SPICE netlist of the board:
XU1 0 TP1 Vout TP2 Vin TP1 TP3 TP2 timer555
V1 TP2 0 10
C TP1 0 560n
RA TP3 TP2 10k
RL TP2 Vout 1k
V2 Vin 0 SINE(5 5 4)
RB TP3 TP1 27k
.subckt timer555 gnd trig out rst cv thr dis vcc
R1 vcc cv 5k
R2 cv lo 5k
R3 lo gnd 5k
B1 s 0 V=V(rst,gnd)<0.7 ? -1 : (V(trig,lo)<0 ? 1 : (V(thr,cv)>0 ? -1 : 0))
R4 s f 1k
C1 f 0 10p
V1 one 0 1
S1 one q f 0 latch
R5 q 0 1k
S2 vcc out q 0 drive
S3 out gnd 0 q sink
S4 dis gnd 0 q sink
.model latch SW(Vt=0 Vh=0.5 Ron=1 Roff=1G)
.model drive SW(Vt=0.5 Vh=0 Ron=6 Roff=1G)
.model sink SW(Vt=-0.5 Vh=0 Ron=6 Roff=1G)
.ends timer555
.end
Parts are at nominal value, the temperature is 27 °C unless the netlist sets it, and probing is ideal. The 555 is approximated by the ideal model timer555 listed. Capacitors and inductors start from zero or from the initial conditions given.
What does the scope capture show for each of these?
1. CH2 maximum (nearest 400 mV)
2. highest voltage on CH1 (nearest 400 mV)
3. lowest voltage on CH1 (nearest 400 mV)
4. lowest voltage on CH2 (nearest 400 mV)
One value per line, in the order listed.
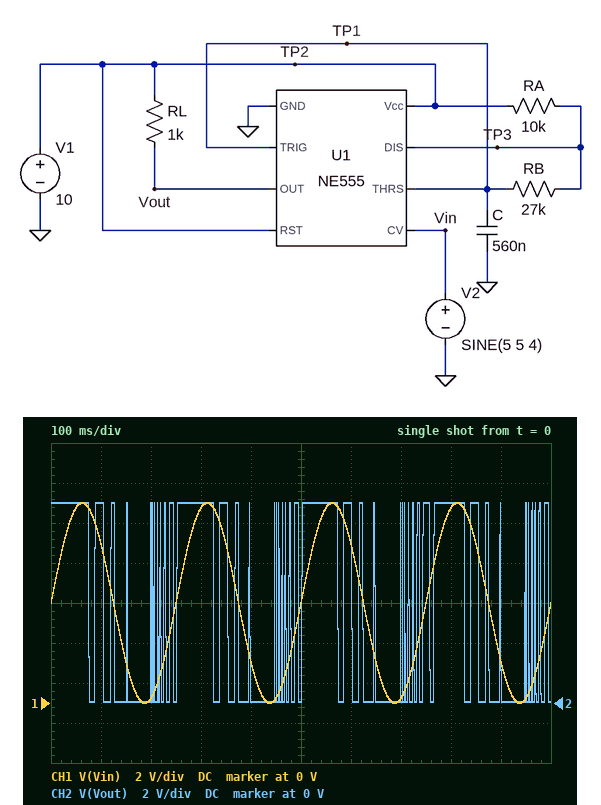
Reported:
10.0 V
10.0 V
0 V
0 V
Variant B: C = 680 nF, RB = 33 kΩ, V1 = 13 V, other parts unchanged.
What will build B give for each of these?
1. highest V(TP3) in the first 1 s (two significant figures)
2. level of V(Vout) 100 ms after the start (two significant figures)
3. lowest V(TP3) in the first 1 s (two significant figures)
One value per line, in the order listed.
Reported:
12 V
13 V
7.8 mV
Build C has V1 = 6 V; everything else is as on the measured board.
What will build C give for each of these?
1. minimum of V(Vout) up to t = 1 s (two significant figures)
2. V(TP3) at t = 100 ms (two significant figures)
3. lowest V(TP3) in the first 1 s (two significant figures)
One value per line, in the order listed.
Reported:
36 mV
6.0 V
3.6 mV
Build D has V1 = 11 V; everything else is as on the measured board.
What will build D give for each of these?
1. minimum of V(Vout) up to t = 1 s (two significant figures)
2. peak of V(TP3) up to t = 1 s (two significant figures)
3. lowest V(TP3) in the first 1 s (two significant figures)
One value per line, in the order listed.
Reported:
66 mV
11 V
6.6 mV
